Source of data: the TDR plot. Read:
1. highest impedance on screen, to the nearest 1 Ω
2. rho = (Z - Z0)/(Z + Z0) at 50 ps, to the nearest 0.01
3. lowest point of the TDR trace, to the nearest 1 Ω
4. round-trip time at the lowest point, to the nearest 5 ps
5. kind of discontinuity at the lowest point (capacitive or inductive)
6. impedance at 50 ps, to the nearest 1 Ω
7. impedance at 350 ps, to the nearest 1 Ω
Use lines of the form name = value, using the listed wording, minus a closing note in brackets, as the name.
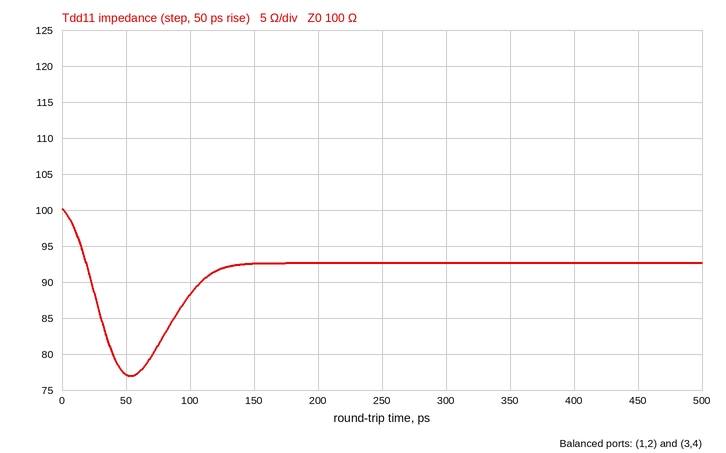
highest impedance on screen, to the nearest 1 Ω = 100 Ω
rho = (Z - Z0)/(Z + Z0) at 50 ps, to the nearest 0.01 = -0.13
lowest point of the TDR trace, to the nearest 1 Ω = 77 Ω
round-trip time at the lowest point, to the nearest 5 ps = 55 ps
kind of discontinuity at the lowest point = capacitive
impedance at 50 ps, to the nearest 1 Ω = 77 Ω
impedance at 350 ps, to the nearest 1 Ω = 93 Ω
